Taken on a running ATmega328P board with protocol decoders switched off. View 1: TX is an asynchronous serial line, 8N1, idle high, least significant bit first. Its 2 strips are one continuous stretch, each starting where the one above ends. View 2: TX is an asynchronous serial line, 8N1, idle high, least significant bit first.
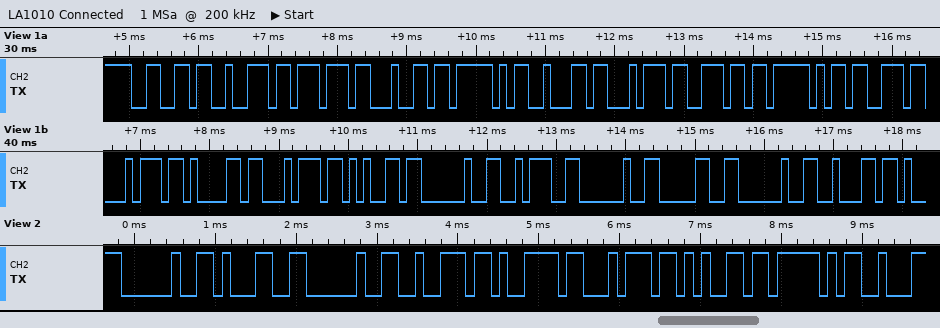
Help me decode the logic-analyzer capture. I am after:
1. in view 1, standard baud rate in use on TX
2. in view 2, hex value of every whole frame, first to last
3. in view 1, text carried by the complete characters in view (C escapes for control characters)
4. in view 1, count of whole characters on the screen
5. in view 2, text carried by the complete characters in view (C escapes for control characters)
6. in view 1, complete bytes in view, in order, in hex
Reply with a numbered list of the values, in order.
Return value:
1. 9600 baud
2. 20 31 20 72 79 74 65 5F
3. "frwd_btn_state : 0 b"
4. 20
5. " 1 ryte_"
6. 66 72 77 64 5F 62 74 6E 5F 73 74 61 74 65 20 3A 20 30 20 62
